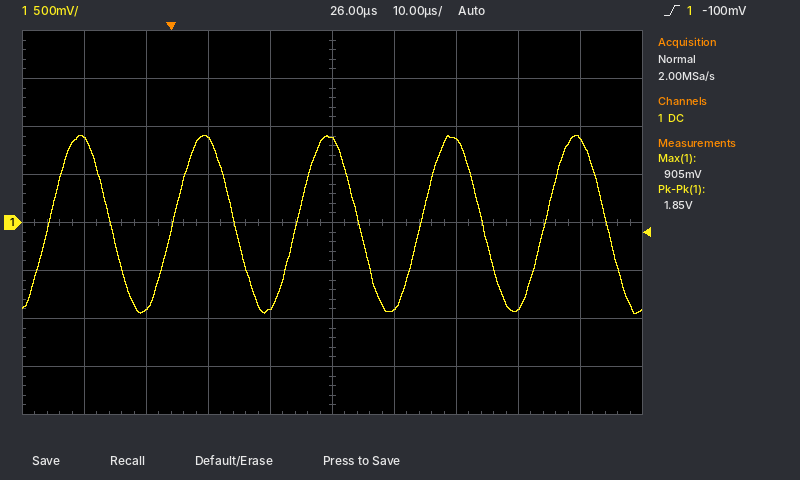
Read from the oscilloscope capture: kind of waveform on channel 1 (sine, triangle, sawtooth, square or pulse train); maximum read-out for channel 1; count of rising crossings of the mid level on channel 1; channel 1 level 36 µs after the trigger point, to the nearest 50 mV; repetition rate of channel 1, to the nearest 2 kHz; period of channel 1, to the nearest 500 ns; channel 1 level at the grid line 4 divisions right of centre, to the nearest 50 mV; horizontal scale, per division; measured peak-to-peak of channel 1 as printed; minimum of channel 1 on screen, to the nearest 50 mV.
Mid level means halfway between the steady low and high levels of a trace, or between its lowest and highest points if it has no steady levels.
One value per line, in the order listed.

sine
905 mV
5
-900 mV
50 kHz
20.0 µs
850 mV
10 µs
1.85 V
-950 mV
